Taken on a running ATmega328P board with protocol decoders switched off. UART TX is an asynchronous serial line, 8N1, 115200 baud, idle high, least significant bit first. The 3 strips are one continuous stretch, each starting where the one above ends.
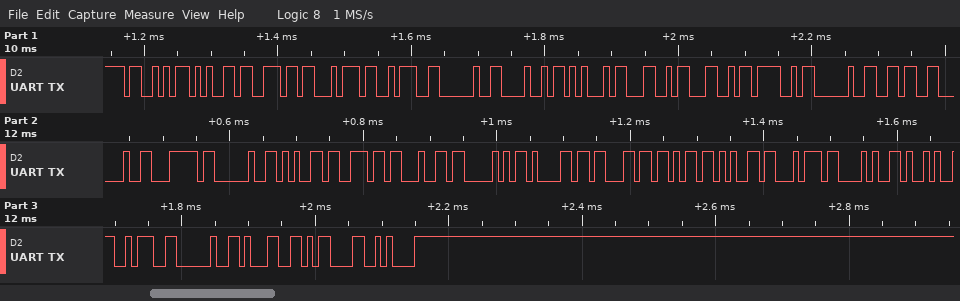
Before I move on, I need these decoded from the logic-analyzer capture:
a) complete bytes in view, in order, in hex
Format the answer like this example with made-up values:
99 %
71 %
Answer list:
0x53 0x65 0x6E 0x74 0x3A 0x20 0x48 0x45 0x4C 0x4C 0x4F 0x20 0x36 0x20 0x7C 0x20 0x65 0x6E 0x64 0x50 0x61 0x63 0x6B 0x65 0x74 0x28 0x29 0x3A 0x20 0x31 0x0D 0x0A
